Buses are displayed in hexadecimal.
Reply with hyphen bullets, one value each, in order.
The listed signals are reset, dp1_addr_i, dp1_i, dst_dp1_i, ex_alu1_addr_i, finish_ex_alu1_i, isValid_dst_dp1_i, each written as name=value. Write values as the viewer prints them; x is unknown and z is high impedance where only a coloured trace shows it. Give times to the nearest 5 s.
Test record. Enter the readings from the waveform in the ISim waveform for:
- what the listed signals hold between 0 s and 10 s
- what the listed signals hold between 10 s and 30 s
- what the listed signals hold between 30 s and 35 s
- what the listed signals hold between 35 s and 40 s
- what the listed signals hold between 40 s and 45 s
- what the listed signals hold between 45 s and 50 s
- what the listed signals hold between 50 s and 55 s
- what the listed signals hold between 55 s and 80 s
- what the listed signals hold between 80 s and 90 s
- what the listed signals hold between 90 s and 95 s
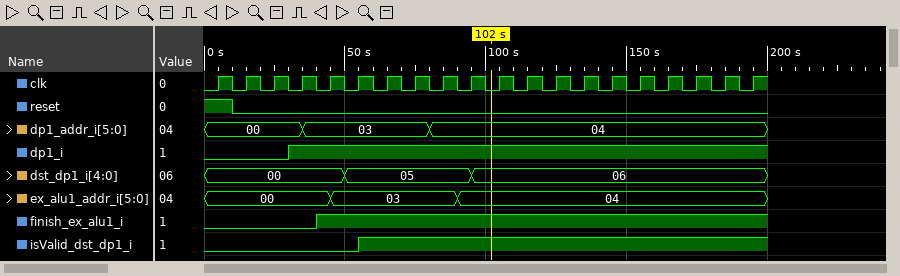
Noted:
- reset=1, dp1_addr_i=00, dp1_i=0, dst_dp1_i=00, ex_alu1_addr_i=00, finish_ex_alu1_i=0, isValid_dst_dp1_i=0
- reset=0, dp1_addr_i=00, dp1_i=0, dst_dp1_i=00, ex_alu1_addr_i=00, finish_ex_alu1_i=0, isValid_dst_dp1_i=0
- reset=0, dp1_addr_i=00, dp1_i=1, dst_dp1_i=00, ex_alu1_addr_i=00, finish_ex_alu1_i=0, isValid_dst_dp1_i=0
- reset=0, dp1_addr_i=03, dp1_i=1, dst_dp1_i=00, ex_alu1_addr_i=00, finish_ex_alu1_i=0, isValid_dst_dp1_i=0
- reset=0, dp1_addr_i=03, dp1_i=1, dst_dp1_i=00, ex_alu1_addr_i=00, finish_ex_alu1_i=1, isValid_dst_dp1_i=0
- reset=0, dp1_addr_i=03, dp1_i=1, dst_dp1_i=00, ex_alu1_addr_i=03, finish_ex_alu1_i=1, isValid_dst_dp1_i=0
- reset=0, dp1_addr_i=03, dp1_i=1, dst_dp1_i=05, ex_alu1_addr_i=03, finish_ex_alu1_i=1, isValid_dst_dp1_i=0
- reset=0, dp1_addr_i=03, dp1_i=1, dst_dp1_i=05, ex_alu1_addr_i=03, finish_ex_alu1_i=1, isValid_dst_dp1_i=1
- reset=0, dp1_addr_i=04, dp1_i=1, dst_dp1_i=05, ex_alu1_addr_i=03, finish_ex_alu1_i=1, isValid_dst_dp1_i=1
- reset=0, dp1_addr_i=04, dp1_i=1, dst_dp1_i=05, ex_alu1_addr_i=04, finish_ex_alu1_i=1, isValid_dst_dp1_i=1
